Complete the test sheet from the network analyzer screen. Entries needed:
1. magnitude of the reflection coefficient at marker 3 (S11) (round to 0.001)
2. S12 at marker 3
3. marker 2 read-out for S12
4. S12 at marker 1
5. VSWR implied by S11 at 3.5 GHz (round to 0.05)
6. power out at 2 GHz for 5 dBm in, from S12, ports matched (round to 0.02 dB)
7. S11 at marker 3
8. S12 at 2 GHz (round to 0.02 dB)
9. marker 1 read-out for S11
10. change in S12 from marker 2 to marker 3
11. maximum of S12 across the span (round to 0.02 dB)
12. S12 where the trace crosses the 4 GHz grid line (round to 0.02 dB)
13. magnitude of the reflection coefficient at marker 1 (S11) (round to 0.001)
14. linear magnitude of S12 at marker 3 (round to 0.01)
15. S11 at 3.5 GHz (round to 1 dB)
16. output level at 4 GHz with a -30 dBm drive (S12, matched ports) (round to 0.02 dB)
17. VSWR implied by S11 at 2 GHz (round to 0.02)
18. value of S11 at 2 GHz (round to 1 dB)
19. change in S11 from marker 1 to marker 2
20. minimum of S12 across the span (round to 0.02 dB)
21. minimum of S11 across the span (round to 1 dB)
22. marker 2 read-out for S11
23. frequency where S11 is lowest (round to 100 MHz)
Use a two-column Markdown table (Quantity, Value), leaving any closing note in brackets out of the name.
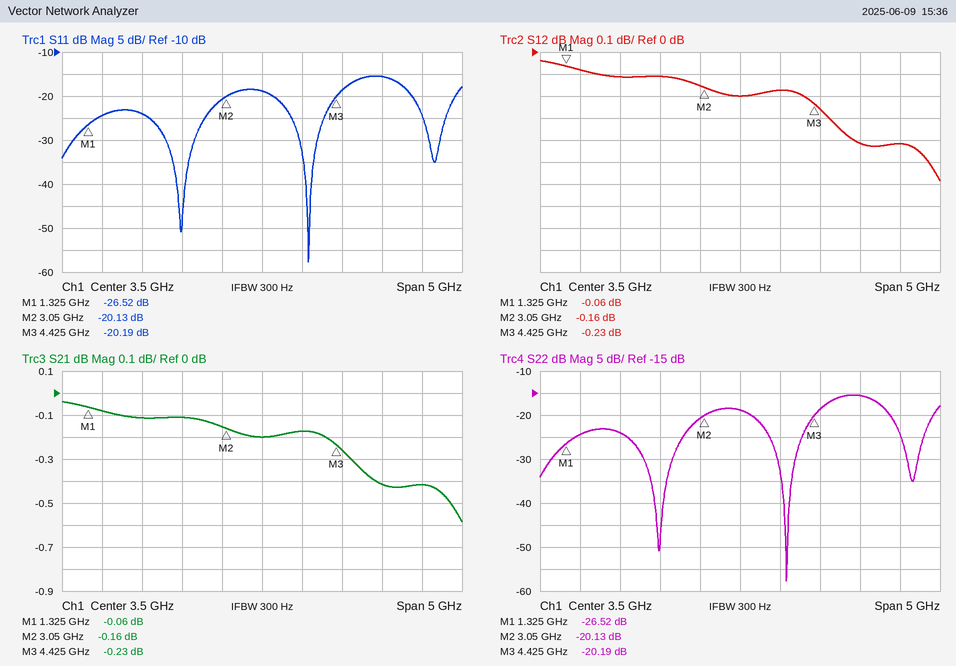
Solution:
| Quantity | Value |
|---|---|
| magnitude of the reflection coefficient at marker 3 (S11) | 0.098 |
| S12 at marker 3 | -0.23 dB |
| marker 2 read-out for S12 | -0.16 dB |
| S12 at marker 1 | -0.06 dB |
| VSWR implied by S11 at 3.5 GHz | 1.25 |
| power out at 2 GHz for 5 dBm in, from S12, ports matched | 4.88 dBm |
| S11 at marker 3 | -20.19 dB |
| S12 at 2 GHz | -0.12 dB |
| marker 1 read-out for S11 | -26.52 dB |
| change in S12 from marker 2 to marker 3 | -0.07 dB |
| maximum of S12 across the span | -0.04 dB |
| S12 where the trace crosses the 4 GHz grid line | -0.18 dB |
| magnitude of the reflection coefficient at marker 1 (S11) | 0.047 |
| linear magnitude of S12 at marker 3 | 0.97 |
| S11 at 3.5 GHz | -19 dB |
| output level at 4 GHz with a -30 dBm drive (S12, matched ports) | -30.18 dBm |
| VSWR implied by S11 at 2 GHz | 1.14 |
| value of S11 at 2 GHz | -24 dB |
| change in S11 from marker 1 to marker 2 | 6.39 dB |
| minimum of S12 across the span | -0.58 dB |
| minimum of S11 across the span | -58 dB |
| marker 2 read-out for S11 | -20.13 dB |
| frequency where S11 is lowest | 4.1 GHz |
